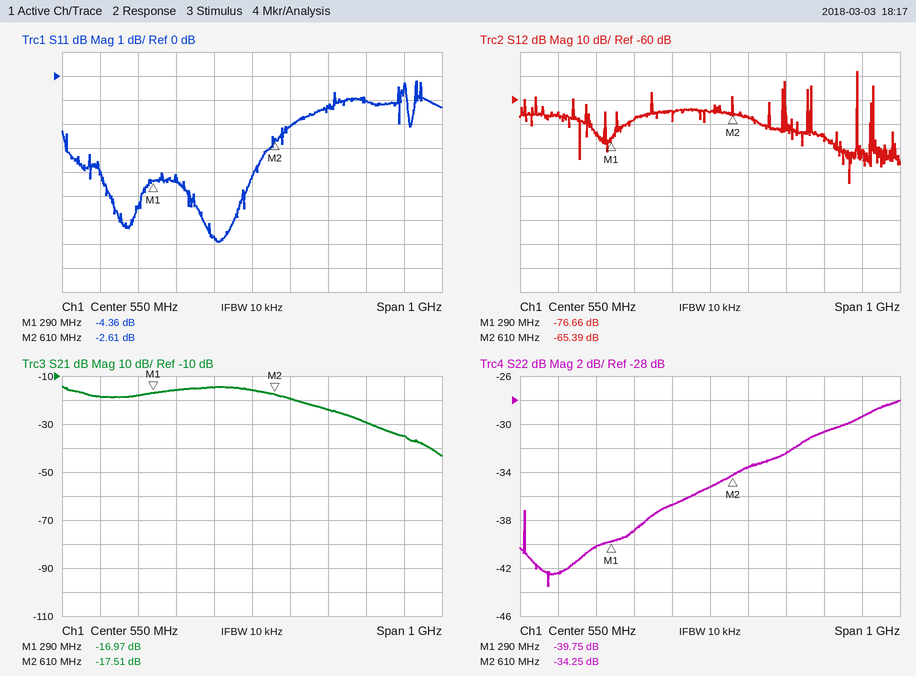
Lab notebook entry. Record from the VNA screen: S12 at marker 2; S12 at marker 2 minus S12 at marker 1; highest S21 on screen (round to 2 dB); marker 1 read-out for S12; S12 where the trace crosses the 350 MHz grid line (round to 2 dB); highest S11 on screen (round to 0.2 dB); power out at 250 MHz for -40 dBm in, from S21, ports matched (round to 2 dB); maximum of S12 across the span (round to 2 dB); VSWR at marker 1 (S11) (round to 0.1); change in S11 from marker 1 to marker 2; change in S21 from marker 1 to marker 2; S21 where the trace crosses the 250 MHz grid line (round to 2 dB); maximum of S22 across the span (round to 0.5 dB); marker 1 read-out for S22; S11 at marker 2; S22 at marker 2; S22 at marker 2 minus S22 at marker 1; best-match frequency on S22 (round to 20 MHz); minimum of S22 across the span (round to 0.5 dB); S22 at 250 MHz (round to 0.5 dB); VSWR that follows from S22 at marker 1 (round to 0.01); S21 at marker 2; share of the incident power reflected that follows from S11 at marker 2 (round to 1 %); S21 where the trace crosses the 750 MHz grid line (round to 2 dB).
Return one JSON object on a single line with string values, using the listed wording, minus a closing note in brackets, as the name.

{"S12 at marker 2": "-65.39 dB", "S12 at marker 2 minus S12 at marker 1": "11.27 dB", "highest S21 on screen": "-14 dB", "marker 1 read-out for S12": "-76.66 dB", "S12 where the trace crosses the 350 MHz grid line": "-68 dB", "highest S11 on screen": "-0.2 dB", "power out at 250 MHz for -40 dBm in, from S21, ports matched": "-58 dBm", "maximum of S12 across the span": "-48 dB", "VSWR at marker 1 (S11)": "4.1", "change in S11 from marker 1 to marker 2": "1.75 dB", "change in S21 from marker 1 to marker 2": "-0.54 dB", "S21 where the trace crosses the 250 MHz grid line": "-18 dB", "maximum of S22 across the span": "-28.0 dB", "marker 1 read-out for S22": "-39.75 dB", "S11 at marker 2": "-2.61 dB", "S22 at marker 2": "-34.25 dB", "S22 at marker 2 minus S22 at marker 1": "5.50 dB", "best-match frequency on S22": "120 MHz", "minimum of S22 across the span": "-43.5 dB", "S22 at 250 MHz": "-40.0 dB", "VSWR that follows from S22 at marker 1": "1.02", "S21 at marker 2": "-17.51 dB", "share of the incident power reflected that follows from S11 at marker 2": "55 %", "S21 where the trace crosses the 750 MHz grid line": "-24 dB"}
